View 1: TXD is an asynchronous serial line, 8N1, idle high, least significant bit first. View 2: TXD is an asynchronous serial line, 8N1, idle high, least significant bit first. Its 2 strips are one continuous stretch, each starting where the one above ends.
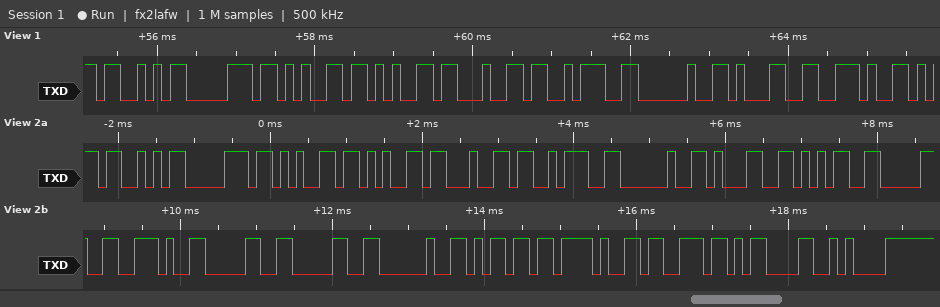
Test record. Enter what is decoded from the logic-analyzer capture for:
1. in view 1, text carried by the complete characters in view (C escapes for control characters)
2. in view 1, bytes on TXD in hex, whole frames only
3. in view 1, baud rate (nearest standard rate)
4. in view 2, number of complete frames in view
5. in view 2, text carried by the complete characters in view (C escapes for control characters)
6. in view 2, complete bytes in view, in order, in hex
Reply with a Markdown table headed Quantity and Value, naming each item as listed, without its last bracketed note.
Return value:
| Quantity | Value |
|---|---|
| in view 1, text carried by the complete characters in view | "Speed: 1." |
| in view 1, bytes on TXD in hex, whole frames only | 53 70 65 65 64 3A 20 31 2E |
| in view 1, baud rate | 9600 baud |
| in view 2, number of complete frames in view | 19 |
| in view 2, text carried by the complete characters in view | "Speed: 150.00 m/s\r\n" |
| in view 2, complete bytes in view, in order, in hex | 53 70 65 65 64 3A 20 31 35 30 2E 30 30 20 6D 2F 73 0D 0A |
